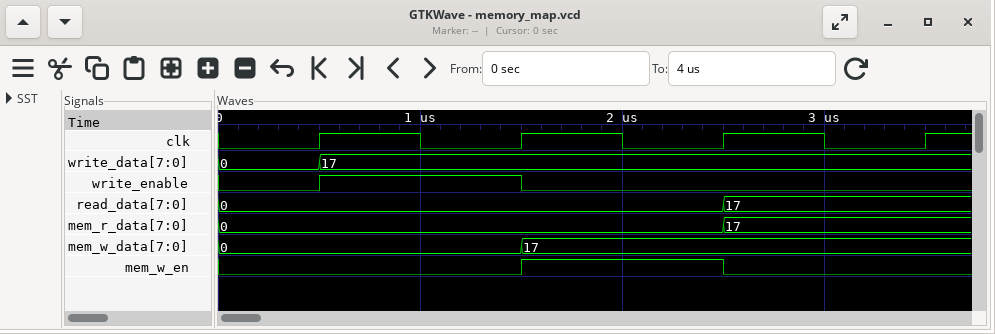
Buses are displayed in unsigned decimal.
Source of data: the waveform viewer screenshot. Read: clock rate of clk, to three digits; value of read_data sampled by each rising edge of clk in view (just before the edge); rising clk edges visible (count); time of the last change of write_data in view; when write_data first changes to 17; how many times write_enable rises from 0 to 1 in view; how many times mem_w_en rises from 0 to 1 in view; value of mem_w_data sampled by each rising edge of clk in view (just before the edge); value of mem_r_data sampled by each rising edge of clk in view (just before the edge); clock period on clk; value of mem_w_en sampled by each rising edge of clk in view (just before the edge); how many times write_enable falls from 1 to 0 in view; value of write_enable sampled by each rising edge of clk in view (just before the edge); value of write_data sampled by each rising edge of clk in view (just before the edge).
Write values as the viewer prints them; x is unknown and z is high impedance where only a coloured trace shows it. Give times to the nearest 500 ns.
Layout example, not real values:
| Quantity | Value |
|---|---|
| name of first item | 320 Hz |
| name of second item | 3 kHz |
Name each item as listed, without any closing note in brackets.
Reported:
| Quantity | Value |
|---|---|
| clock rate of clk, to three digits | 1.00 MHz |
| value of read_data sampled by each rising edge of clk in view | 0, 0, 0, 17 |
| rising clk edges visible | 4 |
| time of the last change of write_data in view | 500 ns |
| when write_data first changes to 17 | 500 ns |
| how many times write_enable rises from 0 to 1 in view | 1 |
| how many times mem_w_en rises from 0 to 1 in view | 1 |
| value of mem_w_data sampled by each rising edge of clk in view | 0, 0, 17, 17 |
| value of mem_r_data sampled by each rising edge of clk in view | 0, 0, 0, 17 |
| clock period on clk | 1000 ns |
| value of mem_w_en sampled by each rising edge of clk in view | 0 0 1 0 |
| how many times write_enable falls from 1 to 0 in view | 1 |
| value of write_enable sampled by each rising edge of clk in view | 0 1 0 0 |
| value of write_data sampled by each rising edge of clk in view | 0, 17, 17, 17 |
